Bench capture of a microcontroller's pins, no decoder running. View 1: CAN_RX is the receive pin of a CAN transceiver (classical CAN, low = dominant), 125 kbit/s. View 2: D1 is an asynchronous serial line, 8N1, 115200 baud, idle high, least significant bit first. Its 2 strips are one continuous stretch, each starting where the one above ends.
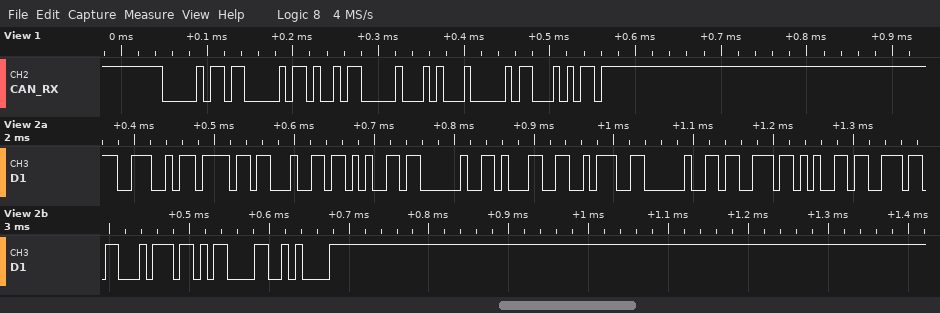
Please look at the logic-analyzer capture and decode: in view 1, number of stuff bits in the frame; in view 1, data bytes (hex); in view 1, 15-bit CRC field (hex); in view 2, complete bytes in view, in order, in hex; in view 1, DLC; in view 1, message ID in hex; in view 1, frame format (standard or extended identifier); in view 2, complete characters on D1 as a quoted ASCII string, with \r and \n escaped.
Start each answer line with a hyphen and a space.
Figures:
- 4
- 4B 00 A2
- 0x0315
- 4E 6F 64 65 20 31 3A 20 73 65 6E 74 0D 0A
- 3
- 0x036
- standard
- "Node 1: sent\r\n"
